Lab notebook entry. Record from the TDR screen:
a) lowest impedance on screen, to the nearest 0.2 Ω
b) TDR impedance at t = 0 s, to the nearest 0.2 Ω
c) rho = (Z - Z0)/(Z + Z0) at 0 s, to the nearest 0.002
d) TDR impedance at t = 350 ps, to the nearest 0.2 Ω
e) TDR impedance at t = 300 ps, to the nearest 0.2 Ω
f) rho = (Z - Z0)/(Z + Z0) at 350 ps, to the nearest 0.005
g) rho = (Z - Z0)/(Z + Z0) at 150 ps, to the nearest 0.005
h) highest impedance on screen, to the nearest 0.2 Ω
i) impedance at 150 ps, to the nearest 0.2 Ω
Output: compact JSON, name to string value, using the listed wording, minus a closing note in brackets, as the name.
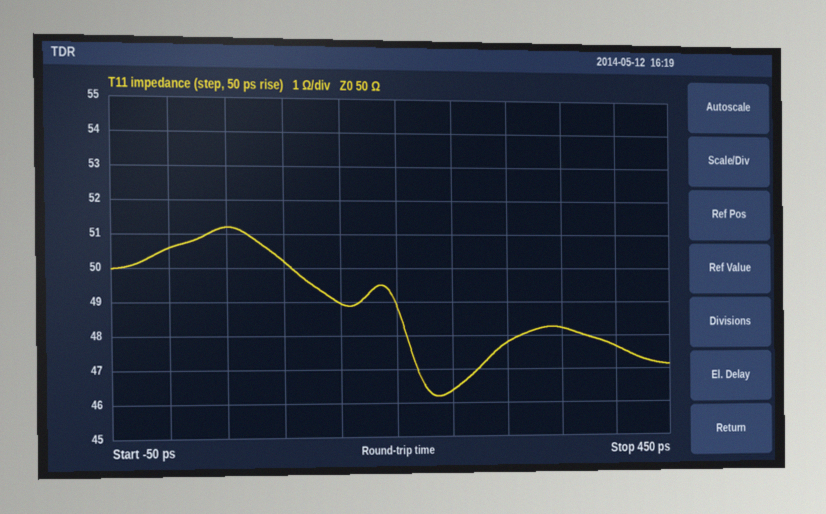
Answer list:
{"lowest impedance on screen, to the nearest 0.2 Ω": "46.2 Ω", "TDR impedance at t = 0 s, to the nearest 0.2 Ω": "50.6 Ω", "rho = (Z - Z0)/(Z + Z0) at 0 s, to the nearest 0.002": "+0.006", "TDR impedance at t = 350 ps, to the nearest 0.2 Ω": "48.2 Ω", "TDR impedance at t = 300 ps, to the nearest 0.2 Ω": "47.8 Ω", "rho = (Z - Z0)/(Z + Z0) at 350 ps, to the nearest 0.005": "-0.020", "rho = (Z - Z0)/(Z + Z0) at 150 ps, to the nearest 0.005": "-0.010", "highest impedance on screen, to the nearest 0.2 Ω": "51.2 Ω", "impedance at 150 ps, to the nearest 0.2 Ω": "49.0 Ω"}
